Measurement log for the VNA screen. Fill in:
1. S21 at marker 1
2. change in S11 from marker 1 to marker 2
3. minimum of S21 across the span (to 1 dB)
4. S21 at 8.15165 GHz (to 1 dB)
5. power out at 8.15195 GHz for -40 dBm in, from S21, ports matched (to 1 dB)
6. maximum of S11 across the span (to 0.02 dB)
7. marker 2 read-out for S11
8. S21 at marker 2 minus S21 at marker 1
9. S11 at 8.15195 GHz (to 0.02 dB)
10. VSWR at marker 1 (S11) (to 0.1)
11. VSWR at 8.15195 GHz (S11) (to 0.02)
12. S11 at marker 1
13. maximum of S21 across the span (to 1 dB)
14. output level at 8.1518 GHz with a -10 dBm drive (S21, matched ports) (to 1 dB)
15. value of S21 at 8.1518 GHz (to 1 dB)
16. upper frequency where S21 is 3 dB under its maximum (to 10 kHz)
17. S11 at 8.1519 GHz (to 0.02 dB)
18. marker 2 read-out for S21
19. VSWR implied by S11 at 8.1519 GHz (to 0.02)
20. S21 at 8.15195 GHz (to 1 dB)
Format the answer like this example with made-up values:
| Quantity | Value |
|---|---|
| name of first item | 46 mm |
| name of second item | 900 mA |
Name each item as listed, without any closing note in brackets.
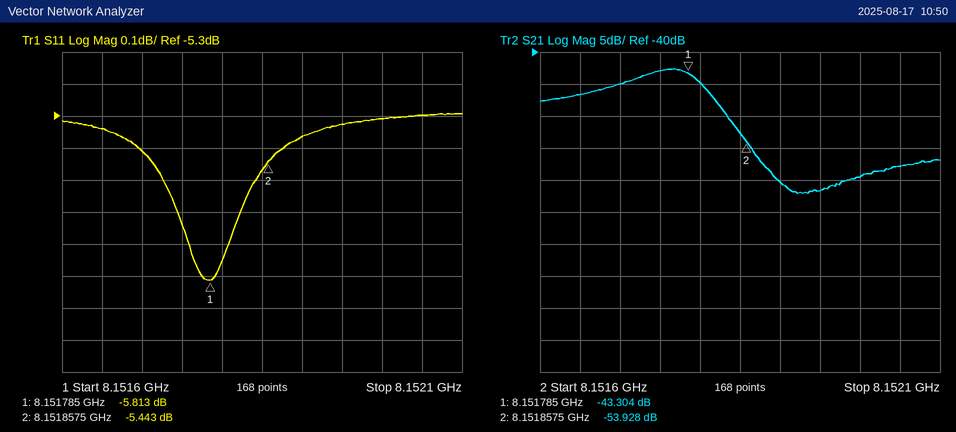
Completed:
| Quantity | Value |
|---|---|
| S21 at marker 1 | -43.304 dB |
| change in S11 from marker 1 to marker 2 | 0.370 dB |
| minimum of S21 across the span | -62 dB |
| S21 at 8.15165 GHz | -47 dB |
| power out at 8.15195 GHz for -40 dBm in, from S21, ports matched | -102 dBm |
| maximum of S11 across the span | -5.30 dB |
| marker 2 read-out for S11 | -5.443 dB |
| S21 at marker 2 minus S21 at marker 1 | -10.624 dB |
| S11 at 8.15195 GHz | -5.32 dB |
| VSWR at marker 1 (S11) | 3.1 |
| VSWR at 8.15195 GHz (S11) | 3.36 |
| S11 at marker 1 | -5.813 dB |
| maximum of S21 across the span | -43 dB |
| output level at 8.1518 GHz with a -10 dBm drive (S21, matched ports) | -55 dBm |
| value of S21 at 8.1518 GHz | -45 dB |
| upper frequency where S21 is 3 dB under its maximum | 8.15181 GHz |
| S11 at 8.1519 GHz | -5.36 dB |
| marker 2 read-out for S21 | -53.928 dB |
| VSWR implied by S11 at 8.1519 GHz | 3.34 |
| S21 at 8.15195 GHz | -62 dB |
